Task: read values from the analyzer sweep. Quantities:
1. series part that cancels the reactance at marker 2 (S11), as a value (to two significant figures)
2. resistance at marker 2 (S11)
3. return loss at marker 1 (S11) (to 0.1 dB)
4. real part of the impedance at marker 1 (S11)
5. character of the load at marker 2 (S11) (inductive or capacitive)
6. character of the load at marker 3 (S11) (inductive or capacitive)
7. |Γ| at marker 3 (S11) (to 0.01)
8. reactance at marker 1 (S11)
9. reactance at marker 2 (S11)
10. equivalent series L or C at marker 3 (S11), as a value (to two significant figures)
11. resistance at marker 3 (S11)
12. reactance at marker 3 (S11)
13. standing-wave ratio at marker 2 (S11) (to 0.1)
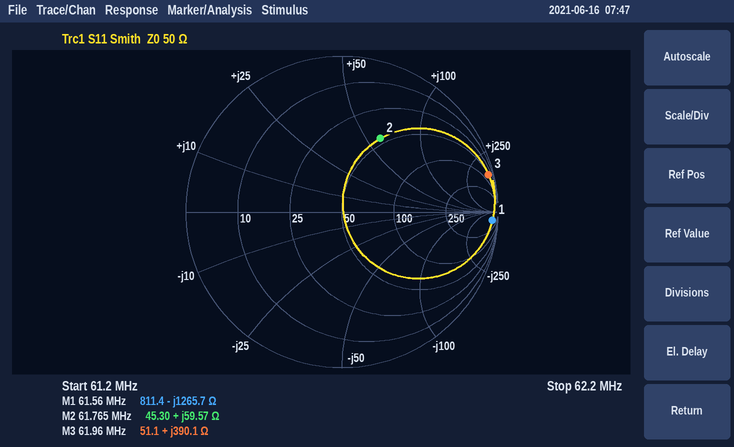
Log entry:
43 pF
45.30 Ω
0.3 dB
811.4 Ω
inductive
inductive
0.97
-1265.7 Ω
+59.57 Ω
1.0 µH
51.1 Ω
+390.1 Ω
3.3
